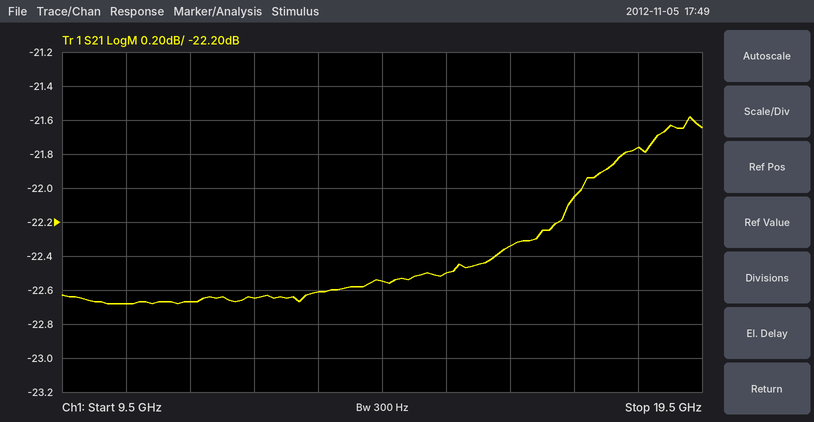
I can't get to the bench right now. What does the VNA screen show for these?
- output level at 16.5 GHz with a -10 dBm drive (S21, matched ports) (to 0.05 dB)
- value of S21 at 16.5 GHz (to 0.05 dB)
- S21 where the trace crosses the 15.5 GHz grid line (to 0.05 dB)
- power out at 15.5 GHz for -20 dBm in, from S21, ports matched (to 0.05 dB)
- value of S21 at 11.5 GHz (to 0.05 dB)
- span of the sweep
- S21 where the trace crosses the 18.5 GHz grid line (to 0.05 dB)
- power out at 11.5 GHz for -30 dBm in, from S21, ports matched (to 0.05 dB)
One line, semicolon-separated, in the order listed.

-32.35 dBm; -22.35 dB; -22.50 dB; -42.50 dBm; -22.65 dB; 10 GHz; -21.75 dB; -52.65 dBm
